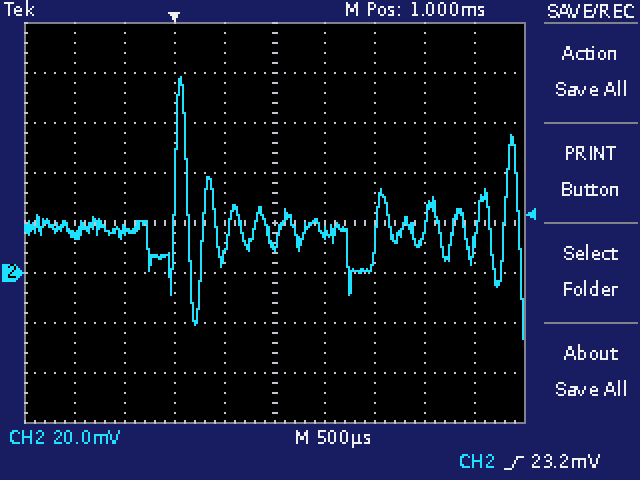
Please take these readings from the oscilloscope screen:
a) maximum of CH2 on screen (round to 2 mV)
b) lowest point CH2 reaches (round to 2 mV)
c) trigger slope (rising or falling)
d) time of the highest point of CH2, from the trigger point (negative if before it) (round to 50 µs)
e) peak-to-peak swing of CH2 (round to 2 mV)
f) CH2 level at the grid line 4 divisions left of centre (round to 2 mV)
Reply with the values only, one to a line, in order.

78 mV
-26 mV
rising
+50 µs
104 mV
16 mV
